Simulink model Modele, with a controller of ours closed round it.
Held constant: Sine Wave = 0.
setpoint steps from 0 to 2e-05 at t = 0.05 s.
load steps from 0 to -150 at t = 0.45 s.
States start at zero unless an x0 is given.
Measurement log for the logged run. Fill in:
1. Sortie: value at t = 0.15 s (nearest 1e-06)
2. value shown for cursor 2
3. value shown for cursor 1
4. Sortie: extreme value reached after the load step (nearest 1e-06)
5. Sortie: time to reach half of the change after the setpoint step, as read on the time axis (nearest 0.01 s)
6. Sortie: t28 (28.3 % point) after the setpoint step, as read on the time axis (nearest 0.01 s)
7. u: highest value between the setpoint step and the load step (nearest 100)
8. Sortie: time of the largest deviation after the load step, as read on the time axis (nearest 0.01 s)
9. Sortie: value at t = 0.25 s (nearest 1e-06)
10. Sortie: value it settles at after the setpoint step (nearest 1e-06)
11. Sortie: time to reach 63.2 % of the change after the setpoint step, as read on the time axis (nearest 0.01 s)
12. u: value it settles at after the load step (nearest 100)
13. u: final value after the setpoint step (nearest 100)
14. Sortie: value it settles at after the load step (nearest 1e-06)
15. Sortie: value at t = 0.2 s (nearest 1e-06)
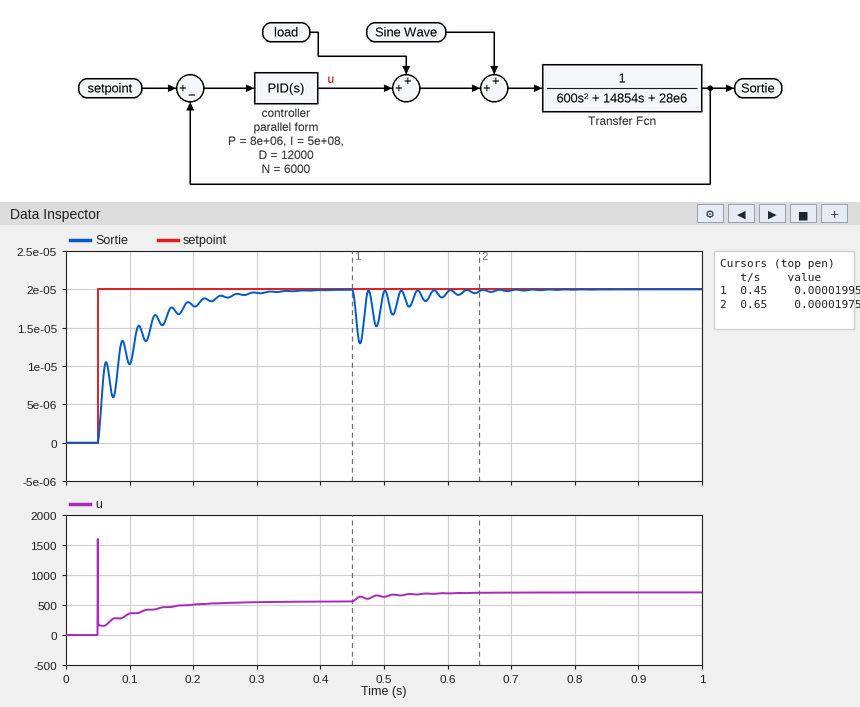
0.000015
0.00001975
0.00001995
0.000013
0.06 s
0.06 s
1600
0.46 s
0.000019
0.000020
0.09 s
700
600
0.000020
0.000018
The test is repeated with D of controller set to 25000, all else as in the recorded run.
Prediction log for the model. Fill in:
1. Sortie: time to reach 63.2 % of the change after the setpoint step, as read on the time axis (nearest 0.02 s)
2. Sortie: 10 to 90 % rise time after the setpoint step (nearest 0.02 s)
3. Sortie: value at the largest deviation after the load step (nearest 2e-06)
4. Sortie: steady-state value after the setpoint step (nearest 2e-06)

0.10 s
0.14 s
0.000014
0.000020
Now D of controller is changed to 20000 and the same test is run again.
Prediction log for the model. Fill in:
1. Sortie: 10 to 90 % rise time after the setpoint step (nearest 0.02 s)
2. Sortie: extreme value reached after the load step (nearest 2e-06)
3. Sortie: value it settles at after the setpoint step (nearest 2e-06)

0.14 s
0.000014
0.000020
